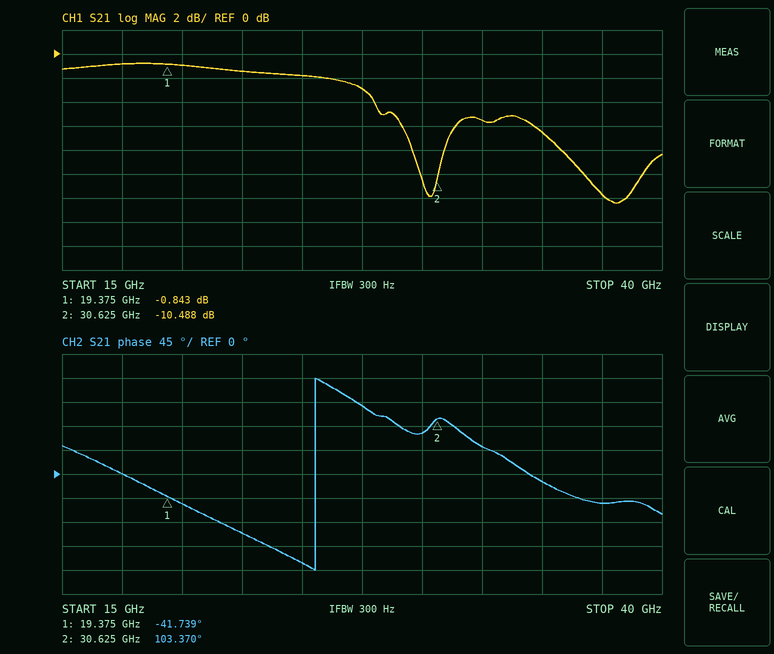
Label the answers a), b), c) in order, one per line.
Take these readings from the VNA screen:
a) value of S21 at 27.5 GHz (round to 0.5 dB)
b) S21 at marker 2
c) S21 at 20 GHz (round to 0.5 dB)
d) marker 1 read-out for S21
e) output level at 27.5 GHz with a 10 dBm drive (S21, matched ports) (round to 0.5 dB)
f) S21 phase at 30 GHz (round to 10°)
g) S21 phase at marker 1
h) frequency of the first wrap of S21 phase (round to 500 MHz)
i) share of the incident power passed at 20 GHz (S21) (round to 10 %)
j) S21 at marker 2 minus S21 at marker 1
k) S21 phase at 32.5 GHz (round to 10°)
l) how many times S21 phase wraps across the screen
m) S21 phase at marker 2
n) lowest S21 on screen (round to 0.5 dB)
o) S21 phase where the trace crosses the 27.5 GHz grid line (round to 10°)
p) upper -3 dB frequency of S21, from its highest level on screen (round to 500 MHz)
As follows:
a) -3.0 dB
b) -10.488 dB
c) -1.0 dB
d) -0.843 dB
e) 7.0 dBm
f) 80°
g) -41.739°
h) 25.5 GHz
i) 80 %
j) -9.645 dB
k) 50°
l) 1
m) 103.370°
n) -12.5 dB
o) 130°
p) 28.0 GHz
